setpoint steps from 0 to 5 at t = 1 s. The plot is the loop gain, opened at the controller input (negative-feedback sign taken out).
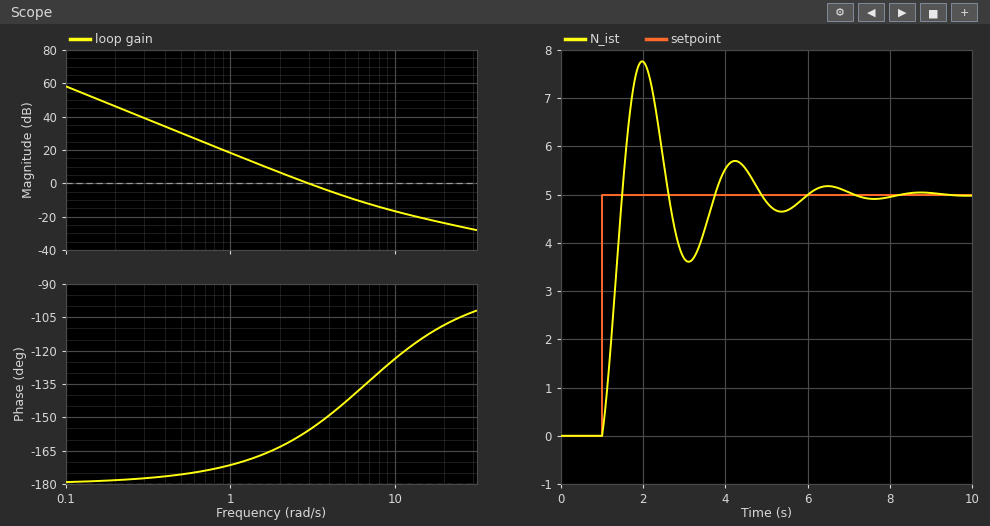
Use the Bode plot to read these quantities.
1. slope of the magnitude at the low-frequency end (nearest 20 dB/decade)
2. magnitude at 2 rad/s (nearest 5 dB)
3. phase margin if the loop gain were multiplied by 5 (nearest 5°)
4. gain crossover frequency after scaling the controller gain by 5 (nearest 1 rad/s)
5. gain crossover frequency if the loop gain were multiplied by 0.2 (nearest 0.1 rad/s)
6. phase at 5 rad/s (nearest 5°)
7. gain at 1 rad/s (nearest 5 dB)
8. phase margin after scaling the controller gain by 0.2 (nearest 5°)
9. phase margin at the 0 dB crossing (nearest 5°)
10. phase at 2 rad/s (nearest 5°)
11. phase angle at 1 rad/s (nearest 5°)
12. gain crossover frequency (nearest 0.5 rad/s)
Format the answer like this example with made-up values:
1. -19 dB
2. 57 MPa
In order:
1. -40 dB/decade
2. 5 dB
3. 50°
4. 8 rad/s
5. 1.3 rad/s
6. -145°
7. 20 dB
8. 10°
9. 25°
10. -165°
11. -170°
12. 3.0 rad/s
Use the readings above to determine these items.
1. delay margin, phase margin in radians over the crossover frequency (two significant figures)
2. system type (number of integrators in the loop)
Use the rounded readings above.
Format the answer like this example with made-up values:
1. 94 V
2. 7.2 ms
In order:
1. 0.15 s
2. 2
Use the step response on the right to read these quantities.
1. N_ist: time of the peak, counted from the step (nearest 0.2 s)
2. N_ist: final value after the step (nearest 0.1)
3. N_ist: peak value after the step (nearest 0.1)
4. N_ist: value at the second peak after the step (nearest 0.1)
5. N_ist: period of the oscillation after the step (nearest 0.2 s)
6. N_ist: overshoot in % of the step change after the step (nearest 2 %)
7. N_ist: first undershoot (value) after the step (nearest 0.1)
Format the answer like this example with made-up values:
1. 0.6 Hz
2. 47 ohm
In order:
1. 1.0 s
2. 5.0
3. 7.8
4. 5.7
5. 2.2 s
6. 56 %
7. 3.6
